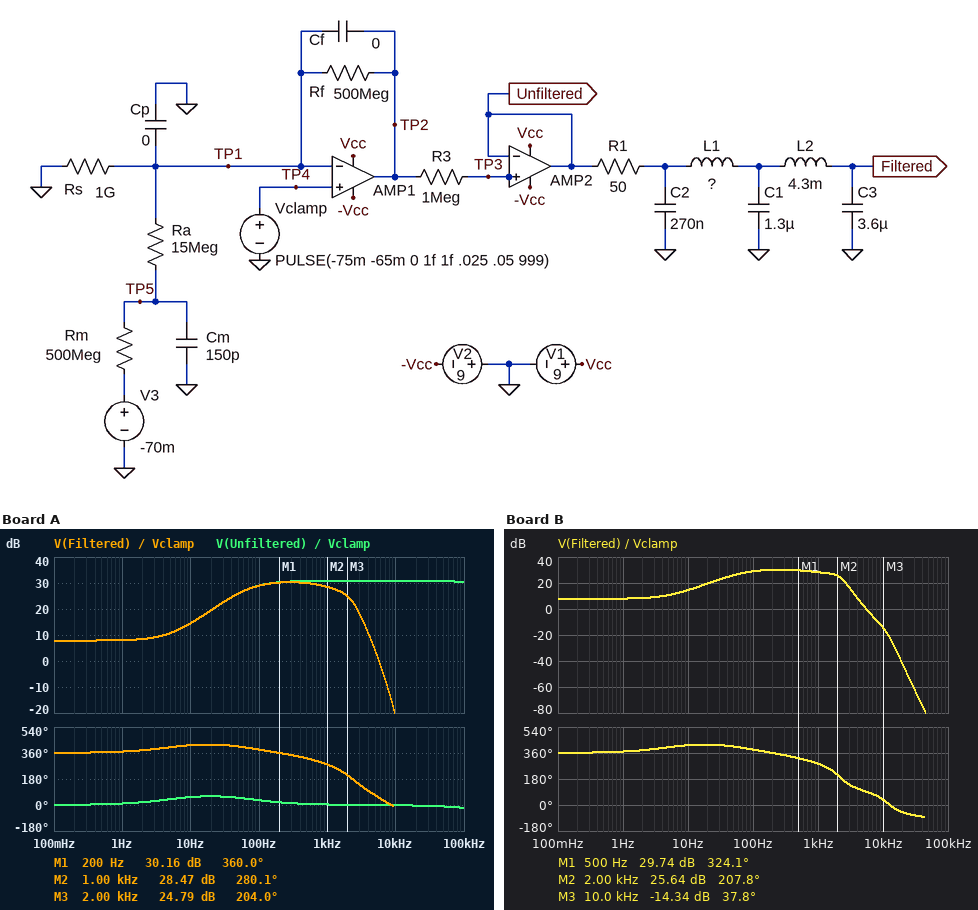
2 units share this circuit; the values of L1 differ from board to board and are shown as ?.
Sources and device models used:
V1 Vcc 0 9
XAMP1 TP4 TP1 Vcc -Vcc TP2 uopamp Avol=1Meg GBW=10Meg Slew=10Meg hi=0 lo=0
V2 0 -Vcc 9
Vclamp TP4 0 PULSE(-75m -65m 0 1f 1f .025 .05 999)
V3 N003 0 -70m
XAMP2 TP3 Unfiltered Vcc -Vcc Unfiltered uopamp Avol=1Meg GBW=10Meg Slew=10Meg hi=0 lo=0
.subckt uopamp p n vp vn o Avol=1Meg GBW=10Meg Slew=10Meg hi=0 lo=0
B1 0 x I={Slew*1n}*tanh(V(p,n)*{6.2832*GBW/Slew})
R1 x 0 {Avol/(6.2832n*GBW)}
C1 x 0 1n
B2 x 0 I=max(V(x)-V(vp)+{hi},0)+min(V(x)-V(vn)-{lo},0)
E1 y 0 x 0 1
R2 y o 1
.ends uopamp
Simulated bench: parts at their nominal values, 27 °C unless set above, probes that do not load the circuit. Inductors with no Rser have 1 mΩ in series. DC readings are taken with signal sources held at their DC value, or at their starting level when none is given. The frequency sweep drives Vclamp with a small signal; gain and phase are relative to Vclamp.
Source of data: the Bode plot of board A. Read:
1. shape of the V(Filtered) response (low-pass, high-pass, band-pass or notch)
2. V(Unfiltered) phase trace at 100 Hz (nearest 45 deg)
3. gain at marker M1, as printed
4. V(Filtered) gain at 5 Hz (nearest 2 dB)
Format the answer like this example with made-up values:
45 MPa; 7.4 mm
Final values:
band-pass; 45 deg; 30.16 dB; 10 dB
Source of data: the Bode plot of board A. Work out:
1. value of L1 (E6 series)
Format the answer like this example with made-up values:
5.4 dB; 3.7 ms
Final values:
1.5 mH
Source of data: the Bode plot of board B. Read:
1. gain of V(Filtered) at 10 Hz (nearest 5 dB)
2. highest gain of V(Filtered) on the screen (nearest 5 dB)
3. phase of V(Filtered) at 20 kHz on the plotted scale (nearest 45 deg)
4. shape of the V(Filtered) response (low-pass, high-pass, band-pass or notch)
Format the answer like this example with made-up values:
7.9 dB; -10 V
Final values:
15 dB; 30 dB; -45 deg; band-pass
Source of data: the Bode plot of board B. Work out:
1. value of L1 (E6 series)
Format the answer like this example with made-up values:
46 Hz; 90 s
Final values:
680 µH
